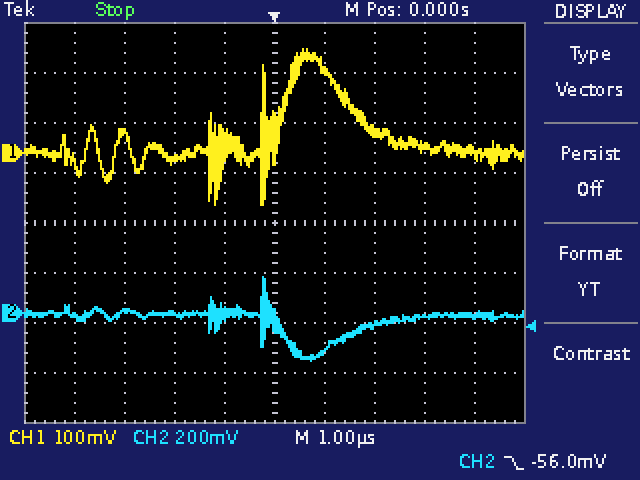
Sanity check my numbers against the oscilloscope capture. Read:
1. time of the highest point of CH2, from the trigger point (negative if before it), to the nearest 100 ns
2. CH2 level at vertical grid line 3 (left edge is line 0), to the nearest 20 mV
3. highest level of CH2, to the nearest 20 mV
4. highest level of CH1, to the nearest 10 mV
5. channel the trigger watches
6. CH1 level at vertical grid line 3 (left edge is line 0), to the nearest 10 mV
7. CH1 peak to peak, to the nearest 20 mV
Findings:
-200 ns
0 mV
140 mV
210 mV
CH2
-10 mV
320 mV
